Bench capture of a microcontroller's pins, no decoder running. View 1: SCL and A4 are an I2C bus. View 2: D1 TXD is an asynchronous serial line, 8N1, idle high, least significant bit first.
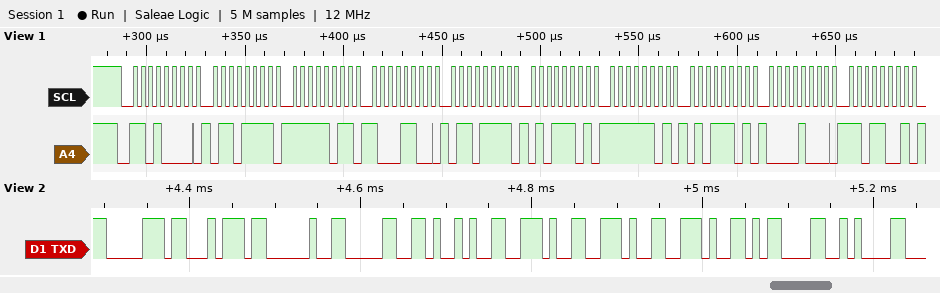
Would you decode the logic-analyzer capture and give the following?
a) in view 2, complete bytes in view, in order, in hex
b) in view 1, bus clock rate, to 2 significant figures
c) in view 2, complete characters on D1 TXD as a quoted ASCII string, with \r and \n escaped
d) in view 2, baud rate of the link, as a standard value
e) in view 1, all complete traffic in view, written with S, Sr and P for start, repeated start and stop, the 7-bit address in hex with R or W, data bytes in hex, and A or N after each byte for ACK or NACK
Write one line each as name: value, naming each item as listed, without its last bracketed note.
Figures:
in view 2, complete bytes in view, in order, in hex: 70 74 20 30 29 2E 2E 2E 0D 0A
in view 1, bus clock rate, to 2 significant figures: 250 kHz
in view 2, complete characters on D1 TXD as a quoted ASCII string, with \r and \n escaped: "pt 0)...\r\n"
in view 2, baud rate of the link, as a standard value: 115200 baud
in view 1, all complete traffic in view, written with S, Sr and P for start, repeated start and stop, the 7-bit address in hex with R or W, data bytes in hex, and A or N after each byte for ACK or NACK: S 68W A 6F A FB A 8C A 6F A 5D A FD A 5D A 08 A D9 A
